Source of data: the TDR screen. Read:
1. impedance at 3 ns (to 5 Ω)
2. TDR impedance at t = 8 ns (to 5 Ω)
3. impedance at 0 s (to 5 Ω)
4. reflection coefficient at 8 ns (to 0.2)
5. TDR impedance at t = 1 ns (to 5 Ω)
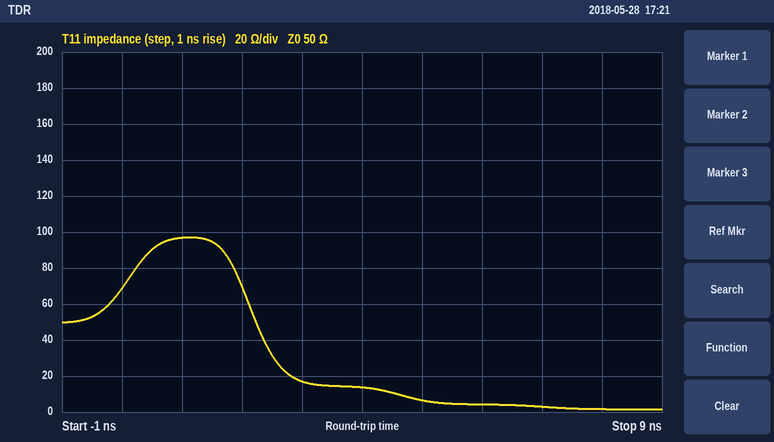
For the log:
15 Ω
0 Ω
70 Ω
-1.0
95 Ω
